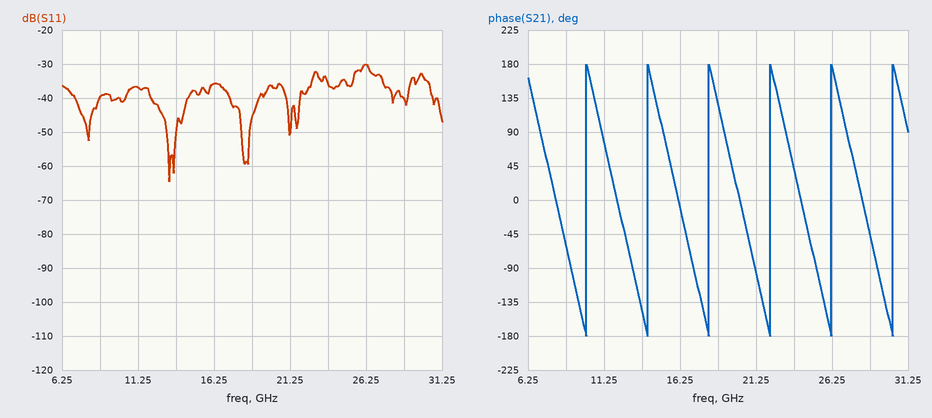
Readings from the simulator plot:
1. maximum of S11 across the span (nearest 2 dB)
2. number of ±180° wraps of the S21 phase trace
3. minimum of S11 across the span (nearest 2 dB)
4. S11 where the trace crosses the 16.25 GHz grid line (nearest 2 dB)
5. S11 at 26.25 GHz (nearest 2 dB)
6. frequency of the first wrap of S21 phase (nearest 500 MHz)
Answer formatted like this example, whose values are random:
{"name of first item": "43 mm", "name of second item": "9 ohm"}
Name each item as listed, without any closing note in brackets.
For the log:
{"maximum of S11 across the span": "-30 dB", "number of ±180° wraps of the S21 phase trace": "6", "minimum of S11 across the span": "-64 dB", "S11 where the trace crosses the 16.25 GHz grid line": "-36 dB", "S11 at 26.25 GHz": "-30 dB", "frequency of the first wrap of S21 phase": "10.0 GHz"}
